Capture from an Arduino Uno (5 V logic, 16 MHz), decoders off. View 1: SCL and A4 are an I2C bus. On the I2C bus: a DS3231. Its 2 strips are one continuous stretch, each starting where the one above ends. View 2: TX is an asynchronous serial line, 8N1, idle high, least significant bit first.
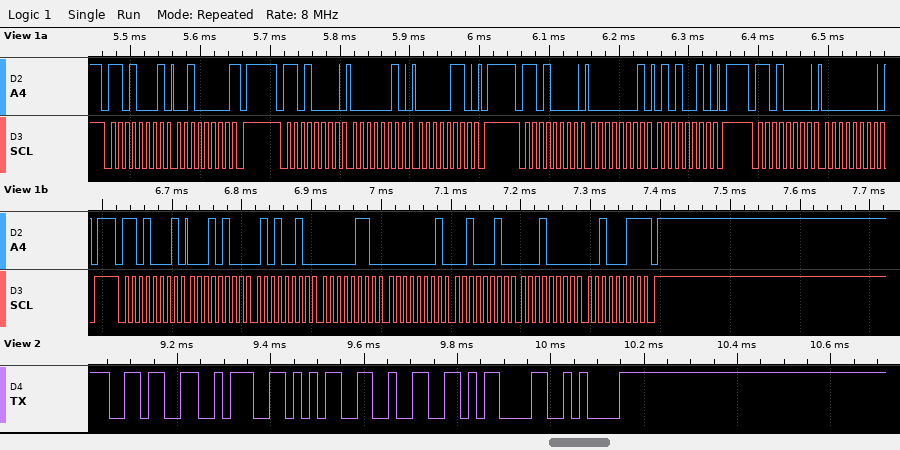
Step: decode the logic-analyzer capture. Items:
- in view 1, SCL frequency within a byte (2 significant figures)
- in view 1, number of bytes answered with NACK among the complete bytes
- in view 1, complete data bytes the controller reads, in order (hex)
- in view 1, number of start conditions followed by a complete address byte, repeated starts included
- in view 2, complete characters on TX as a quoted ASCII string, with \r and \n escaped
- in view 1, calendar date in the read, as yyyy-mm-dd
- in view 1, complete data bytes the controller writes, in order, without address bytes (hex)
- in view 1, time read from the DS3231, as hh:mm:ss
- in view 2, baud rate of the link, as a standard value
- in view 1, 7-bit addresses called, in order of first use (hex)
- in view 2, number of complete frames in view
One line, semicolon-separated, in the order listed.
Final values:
100 kHz; 2; 20 14 52 06 01 22 10 23; 5; "6:52\r\n"; 2023-10-22; 02 06 01 52 00; 06:52:14; 57600 baud; 0x68; 6
